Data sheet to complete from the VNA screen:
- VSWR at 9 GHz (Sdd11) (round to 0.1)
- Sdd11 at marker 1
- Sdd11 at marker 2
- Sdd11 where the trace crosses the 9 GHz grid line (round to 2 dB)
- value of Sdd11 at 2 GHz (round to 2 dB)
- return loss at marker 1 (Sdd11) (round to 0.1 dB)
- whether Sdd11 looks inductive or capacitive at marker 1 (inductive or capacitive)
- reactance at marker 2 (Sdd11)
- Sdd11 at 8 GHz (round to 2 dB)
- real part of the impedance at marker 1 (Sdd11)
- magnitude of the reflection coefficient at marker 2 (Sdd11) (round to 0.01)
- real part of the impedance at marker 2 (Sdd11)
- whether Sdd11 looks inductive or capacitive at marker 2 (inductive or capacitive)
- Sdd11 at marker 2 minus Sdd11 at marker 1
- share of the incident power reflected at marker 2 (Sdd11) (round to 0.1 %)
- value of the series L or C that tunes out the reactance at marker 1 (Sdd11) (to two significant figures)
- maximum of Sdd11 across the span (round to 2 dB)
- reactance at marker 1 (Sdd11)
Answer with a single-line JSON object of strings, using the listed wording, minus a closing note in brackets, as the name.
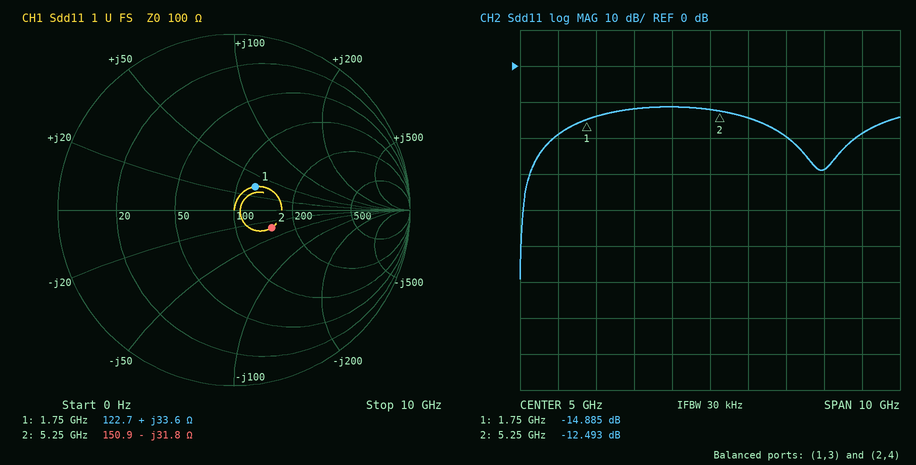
{"VSWR at 9 GHz (Sdd11)": "1.3", "Sdd11 at marker 1": "-14.885 dB", "Sdd11 at marker 2": "-12.493 dB", "Sdd11 where the trace crosses the 9 GHz grid line": "-18 dB", "value of Sdd11 at 2 GHz": "-14 dB", "return loss at marker 1 (Sdd11)": "14.9 dB", "whether Sdd11 looks inductive or capacitive at marker 1": "inductive", "reactance at marker 2": "-31.8 Ω", "Sdd11 at 8 GHz": "-28 dB", "real part of the impedance at marker 1": "122.7 Ω", "magnitude of the reflection coefficient at marker 2 (Sdd11)": "0.24", "real part of the impedance at marker 2": "150.9 Ω", "whether Sdd11 looks inductive or capacitive at marker 2": "capacitive", "Sdd11 at marker 2 minus Sdd11 at marker 1": "2.392 dB", "share of the incident power reflected at marker 2 (Sdd11)": "5.6 %", "value of the series L or C that tunes out the reactance at marker 1 (Sdd11)": "2.7 pF", "maximum of Sdd11 across the span": "-12 dB", "reactance at marker 1": "+33.6 Ω"}
